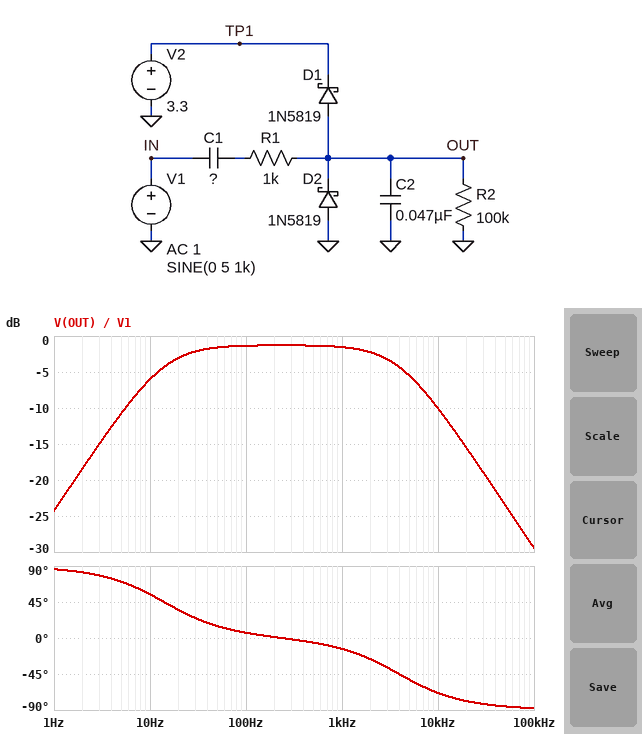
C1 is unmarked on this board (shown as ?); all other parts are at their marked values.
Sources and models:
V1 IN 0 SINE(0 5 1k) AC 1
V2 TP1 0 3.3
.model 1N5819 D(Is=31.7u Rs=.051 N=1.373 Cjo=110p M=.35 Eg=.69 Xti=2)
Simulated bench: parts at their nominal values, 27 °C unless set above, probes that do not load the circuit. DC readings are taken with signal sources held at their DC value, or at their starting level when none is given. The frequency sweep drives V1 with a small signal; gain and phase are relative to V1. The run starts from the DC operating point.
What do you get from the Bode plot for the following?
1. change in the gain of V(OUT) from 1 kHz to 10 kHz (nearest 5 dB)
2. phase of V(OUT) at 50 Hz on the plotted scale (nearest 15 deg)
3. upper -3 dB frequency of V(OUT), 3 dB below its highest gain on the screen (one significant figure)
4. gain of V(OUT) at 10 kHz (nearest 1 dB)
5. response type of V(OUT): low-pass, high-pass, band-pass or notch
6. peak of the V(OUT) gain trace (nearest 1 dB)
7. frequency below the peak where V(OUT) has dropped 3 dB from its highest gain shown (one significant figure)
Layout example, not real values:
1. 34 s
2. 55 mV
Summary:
1. -10 dB
2. 15 deg
3. 4 kHz
4. -10 dB
5. band-pass
6. -1 dB
7. 10 Hz
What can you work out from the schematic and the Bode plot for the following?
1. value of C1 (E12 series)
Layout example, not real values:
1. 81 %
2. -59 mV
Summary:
1. 390 nF
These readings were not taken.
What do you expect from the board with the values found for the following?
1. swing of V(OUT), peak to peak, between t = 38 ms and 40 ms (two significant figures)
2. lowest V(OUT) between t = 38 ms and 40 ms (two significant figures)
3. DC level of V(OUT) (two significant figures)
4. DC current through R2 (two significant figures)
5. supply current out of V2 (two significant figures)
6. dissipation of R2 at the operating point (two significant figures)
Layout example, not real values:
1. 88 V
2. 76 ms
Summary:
1. 3.6 V
2. -160 mV
3. 120 mV
4. 1.2 µA
5. 32 µA
6. 140 nW
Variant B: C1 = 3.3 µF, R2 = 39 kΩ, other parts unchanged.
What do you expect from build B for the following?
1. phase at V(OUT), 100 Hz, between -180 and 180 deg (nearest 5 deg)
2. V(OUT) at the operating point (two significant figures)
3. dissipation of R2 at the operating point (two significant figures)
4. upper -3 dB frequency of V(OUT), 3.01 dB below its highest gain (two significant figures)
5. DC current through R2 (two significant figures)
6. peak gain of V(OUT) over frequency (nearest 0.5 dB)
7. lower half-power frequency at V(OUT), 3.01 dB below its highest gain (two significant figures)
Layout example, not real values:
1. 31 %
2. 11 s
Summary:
1. 0 deg
2. 92 mV
3. 220 nW
4. 3.7 kHz
5. 2.4 µA
6. -1.0 dB
7. 4.0 Hz
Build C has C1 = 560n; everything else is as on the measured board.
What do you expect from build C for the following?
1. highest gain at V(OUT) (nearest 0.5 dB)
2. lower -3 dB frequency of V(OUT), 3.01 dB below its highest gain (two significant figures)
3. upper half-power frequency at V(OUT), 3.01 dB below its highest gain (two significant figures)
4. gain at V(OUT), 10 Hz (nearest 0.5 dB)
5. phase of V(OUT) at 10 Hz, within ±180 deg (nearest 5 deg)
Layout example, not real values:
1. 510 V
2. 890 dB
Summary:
1. -1.0 dB
2. 10 Hz
3. 3.8 kHz
4. -4.0 dB
5. 45 deg
